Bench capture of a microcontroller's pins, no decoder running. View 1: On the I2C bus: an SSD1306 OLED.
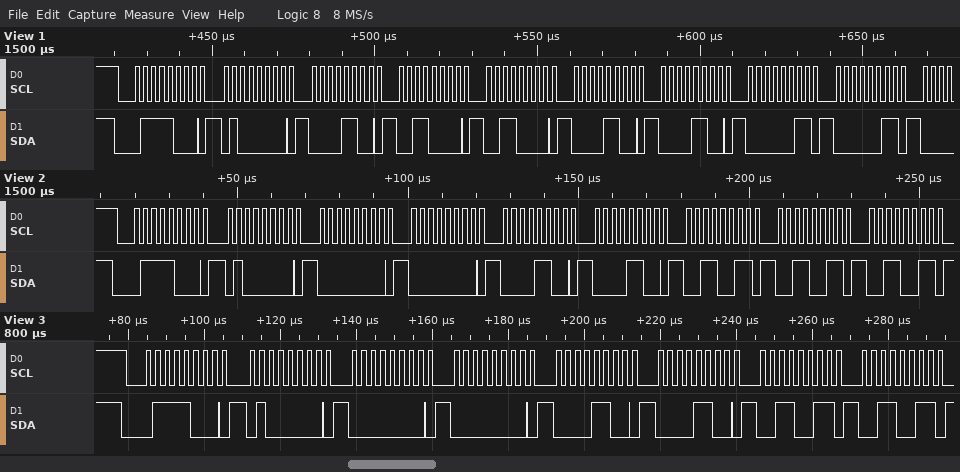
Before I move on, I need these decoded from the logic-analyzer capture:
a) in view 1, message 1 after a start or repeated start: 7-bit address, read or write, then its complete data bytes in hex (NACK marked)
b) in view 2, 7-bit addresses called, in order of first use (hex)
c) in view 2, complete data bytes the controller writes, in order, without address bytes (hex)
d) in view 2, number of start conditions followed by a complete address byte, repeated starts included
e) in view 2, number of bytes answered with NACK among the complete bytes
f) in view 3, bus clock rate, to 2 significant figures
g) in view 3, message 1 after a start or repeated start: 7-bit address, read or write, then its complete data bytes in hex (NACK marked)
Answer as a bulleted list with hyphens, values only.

- 0x3C write: 40 0C 30 30 0C 0C 03 03
- 0x3C
- 40 00 00 0C 0C 33 33 33
- 1
- 0
- 400 kHz
- 0x3C write: 40 00 00 0C 0C 33 33
